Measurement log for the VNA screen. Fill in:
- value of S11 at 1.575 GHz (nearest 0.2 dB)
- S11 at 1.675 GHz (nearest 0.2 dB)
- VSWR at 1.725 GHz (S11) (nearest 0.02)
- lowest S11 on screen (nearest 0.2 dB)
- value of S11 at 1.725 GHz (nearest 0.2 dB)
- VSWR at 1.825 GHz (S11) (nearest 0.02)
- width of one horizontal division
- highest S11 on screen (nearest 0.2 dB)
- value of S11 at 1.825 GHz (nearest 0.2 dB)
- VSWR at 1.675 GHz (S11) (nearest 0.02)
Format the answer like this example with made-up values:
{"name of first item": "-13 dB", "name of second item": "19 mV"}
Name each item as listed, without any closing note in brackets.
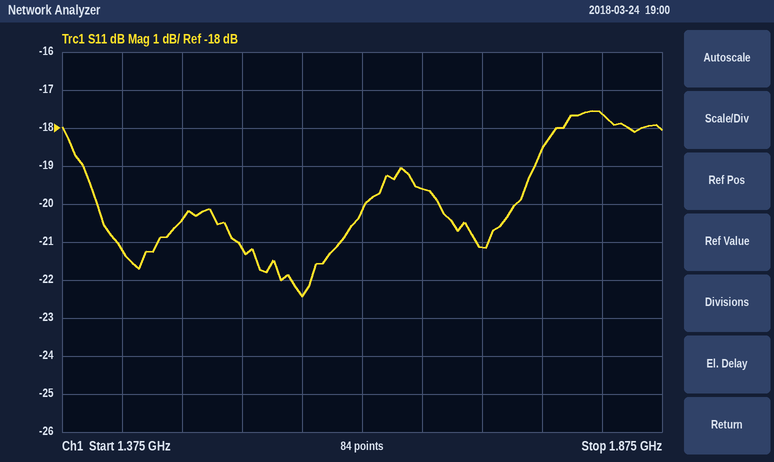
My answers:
{"value of S11 at 1.575 GHz": "-22.4 dB", "S11 at 1.675 GHz": "-19.6 dB", "VSWR at 1.725 GHz (S11)": "1.20", "lowest S11 on screen": "-22.4 dB", "value of S11 at 1.725 GHz": "-21.2 dB", "VSWR at 1.825 GHz (S11)": "1.30", "width of one horizontal division": "50 MHz", "highest S11 on screen": "-17.6 dB", "value of S11 at 1.825 GHz": "-17.6 dB", "VSWR at 1.675 GHz (S11)": "1.24"}
